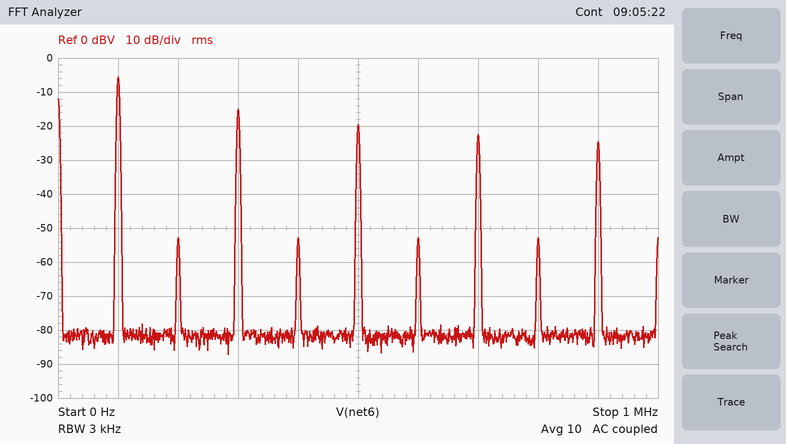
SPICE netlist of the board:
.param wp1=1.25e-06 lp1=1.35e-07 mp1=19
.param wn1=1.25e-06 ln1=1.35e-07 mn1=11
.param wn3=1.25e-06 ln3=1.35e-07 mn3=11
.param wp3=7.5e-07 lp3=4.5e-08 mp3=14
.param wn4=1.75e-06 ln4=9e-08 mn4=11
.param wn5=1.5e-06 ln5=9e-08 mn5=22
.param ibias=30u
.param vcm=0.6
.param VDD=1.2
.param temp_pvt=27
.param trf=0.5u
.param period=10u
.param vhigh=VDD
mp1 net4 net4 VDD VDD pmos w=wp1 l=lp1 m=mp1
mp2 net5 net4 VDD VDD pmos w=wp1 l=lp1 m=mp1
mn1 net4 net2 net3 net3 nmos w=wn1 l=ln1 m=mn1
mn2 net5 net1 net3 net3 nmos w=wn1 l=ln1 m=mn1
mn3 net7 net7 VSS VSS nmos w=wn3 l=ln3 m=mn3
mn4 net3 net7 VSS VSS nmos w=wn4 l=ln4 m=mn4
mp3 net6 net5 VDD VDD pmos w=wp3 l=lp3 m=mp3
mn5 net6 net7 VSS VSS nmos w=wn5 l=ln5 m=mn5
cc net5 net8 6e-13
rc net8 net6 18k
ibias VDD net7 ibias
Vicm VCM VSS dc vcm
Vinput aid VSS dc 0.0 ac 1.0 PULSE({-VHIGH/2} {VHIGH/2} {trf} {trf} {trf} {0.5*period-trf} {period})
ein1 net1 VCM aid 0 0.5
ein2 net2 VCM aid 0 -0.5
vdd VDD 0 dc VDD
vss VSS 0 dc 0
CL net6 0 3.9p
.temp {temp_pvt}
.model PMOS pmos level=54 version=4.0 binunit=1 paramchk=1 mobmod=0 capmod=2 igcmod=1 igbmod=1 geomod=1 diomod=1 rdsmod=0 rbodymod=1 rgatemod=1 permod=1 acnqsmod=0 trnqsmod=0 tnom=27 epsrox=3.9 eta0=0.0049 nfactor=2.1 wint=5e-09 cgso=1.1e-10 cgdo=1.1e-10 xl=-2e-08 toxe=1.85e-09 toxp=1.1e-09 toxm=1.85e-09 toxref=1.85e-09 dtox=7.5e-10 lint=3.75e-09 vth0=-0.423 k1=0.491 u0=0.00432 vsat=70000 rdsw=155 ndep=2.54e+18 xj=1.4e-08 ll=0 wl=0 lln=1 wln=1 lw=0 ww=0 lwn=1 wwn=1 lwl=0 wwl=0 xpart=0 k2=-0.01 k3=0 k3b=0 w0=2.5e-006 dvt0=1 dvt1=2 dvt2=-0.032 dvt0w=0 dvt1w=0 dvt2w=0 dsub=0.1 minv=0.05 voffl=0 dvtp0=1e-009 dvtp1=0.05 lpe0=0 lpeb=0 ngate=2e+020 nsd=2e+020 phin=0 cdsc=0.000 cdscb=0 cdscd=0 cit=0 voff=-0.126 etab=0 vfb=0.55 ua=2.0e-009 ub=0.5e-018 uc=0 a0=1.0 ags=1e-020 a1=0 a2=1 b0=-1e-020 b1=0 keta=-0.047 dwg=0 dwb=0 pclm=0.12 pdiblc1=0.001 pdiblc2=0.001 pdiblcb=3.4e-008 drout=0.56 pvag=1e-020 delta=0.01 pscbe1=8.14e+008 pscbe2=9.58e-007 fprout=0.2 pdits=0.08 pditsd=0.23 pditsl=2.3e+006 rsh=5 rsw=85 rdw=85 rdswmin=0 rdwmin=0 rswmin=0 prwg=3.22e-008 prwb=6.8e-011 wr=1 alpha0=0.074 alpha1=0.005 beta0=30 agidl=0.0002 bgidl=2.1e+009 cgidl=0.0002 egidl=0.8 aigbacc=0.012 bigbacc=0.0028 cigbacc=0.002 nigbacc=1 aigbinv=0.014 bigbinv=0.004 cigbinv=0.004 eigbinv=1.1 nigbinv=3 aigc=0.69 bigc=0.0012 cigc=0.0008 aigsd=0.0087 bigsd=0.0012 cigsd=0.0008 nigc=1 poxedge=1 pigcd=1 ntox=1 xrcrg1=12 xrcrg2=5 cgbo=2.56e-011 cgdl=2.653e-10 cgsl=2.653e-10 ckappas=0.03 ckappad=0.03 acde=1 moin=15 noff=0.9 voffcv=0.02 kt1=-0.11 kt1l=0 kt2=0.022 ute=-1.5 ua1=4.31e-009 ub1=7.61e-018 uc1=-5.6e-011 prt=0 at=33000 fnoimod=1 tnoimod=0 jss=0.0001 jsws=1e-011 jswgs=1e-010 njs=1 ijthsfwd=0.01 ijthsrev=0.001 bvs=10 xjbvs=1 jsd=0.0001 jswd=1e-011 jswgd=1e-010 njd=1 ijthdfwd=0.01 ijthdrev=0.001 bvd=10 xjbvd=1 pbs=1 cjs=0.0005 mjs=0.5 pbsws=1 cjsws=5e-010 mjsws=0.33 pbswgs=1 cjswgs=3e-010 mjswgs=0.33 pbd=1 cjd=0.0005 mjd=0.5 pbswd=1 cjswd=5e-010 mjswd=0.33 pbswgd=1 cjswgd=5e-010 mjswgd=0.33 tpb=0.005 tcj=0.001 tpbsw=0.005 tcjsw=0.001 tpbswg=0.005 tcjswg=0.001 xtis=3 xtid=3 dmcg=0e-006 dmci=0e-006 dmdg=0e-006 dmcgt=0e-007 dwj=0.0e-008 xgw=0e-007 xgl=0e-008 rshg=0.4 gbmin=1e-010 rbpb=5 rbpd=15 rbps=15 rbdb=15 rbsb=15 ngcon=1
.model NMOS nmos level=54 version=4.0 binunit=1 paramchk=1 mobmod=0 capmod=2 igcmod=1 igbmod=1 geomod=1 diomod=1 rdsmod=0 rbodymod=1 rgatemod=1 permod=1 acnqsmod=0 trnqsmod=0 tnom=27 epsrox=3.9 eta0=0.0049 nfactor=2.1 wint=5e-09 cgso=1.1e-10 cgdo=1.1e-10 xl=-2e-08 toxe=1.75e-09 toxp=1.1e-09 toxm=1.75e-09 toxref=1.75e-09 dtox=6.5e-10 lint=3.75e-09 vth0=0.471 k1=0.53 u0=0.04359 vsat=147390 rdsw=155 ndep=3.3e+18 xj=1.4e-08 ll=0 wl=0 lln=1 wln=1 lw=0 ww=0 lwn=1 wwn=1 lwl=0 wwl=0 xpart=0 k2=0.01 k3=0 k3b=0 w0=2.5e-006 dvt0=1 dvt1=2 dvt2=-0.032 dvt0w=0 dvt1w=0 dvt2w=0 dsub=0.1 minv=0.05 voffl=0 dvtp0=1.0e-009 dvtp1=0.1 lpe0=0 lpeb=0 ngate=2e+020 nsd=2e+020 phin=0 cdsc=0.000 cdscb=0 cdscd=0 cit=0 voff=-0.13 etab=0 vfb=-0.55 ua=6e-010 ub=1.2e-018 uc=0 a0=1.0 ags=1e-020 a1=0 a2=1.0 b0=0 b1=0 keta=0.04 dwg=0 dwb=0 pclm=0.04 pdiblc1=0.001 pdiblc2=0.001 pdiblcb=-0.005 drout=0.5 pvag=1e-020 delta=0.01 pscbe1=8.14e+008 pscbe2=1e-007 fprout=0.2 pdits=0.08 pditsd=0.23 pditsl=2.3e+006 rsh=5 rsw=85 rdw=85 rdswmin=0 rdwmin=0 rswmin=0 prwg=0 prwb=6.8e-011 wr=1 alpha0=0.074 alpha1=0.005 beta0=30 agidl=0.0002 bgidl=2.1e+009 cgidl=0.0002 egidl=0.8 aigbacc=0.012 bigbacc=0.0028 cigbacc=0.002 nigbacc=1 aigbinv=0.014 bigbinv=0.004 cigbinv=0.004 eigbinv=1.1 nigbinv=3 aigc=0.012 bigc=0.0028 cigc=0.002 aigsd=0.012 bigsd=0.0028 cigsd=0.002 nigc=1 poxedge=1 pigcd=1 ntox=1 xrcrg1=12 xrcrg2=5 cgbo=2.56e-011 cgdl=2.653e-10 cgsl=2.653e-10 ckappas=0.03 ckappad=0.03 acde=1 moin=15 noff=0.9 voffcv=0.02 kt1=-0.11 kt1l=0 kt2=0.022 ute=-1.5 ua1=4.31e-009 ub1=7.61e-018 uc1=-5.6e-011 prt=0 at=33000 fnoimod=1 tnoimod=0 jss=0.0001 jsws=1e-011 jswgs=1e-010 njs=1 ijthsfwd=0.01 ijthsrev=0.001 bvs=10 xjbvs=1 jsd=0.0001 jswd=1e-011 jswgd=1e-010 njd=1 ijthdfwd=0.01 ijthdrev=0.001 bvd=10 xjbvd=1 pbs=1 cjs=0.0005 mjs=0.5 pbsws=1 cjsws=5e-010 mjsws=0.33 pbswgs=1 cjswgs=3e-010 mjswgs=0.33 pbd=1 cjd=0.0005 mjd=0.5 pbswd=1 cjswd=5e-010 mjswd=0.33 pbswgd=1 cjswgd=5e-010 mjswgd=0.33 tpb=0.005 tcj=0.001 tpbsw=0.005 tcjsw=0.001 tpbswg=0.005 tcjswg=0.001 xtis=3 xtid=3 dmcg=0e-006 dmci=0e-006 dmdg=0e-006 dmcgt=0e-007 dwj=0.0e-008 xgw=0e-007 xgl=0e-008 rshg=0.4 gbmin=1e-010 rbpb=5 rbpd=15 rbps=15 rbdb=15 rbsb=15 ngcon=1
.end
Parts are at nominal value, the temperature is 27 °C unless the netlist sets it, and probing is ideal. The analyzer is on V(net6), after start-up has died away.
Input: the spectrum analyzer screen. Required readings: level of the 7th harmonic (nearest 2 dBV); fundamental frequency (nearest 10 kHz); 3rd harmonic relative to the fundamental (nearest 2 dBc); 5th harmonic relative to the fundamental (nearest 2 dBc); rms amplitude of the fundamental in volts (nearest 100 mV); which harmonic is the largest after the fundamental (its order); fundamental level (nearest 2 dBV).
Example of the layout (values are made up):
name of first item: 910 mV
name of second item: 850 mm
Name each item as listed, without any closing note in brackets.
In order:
level of the 7th harmonic: -22 dBV
fundamental frequency: 100 kHz
3rd harmonic relative to the fundamental: -10 dBc
5th harmonic relative to the fundamental: -14 dBc
rms amplitude of the fundamental in volts: 500 mV
which harmonic is the largest after the fundamental: 3
fundamental level: -6 dBV
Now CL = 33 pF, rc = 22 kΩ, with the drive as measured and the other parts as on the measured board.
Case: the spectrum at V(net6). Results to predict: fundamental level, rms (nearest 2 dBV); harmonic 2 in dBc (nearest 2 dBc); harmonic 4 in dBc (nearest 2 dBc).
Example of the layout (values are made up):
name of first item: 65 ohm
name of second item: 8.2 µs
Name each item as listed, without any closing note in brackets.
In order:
fundamental level, rms: -6 dBV
harmonic 2 in dBc: -28 dBc
harmonic 4 in dBc: -28 dBc
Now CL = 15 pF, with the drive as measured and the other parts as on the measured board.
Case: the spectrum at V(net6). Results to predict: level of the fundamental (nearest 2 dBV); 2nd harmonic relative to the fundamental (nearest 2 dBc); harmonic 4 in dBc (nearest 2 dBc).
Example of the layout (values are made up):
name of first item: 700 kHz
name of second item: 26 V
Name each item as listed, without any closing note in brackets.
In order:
level of the fundamental: -6 dBV
2nd harmonic relative to the fundamental: -36 dBc
harmonic 4 in dBc: -36 dBc
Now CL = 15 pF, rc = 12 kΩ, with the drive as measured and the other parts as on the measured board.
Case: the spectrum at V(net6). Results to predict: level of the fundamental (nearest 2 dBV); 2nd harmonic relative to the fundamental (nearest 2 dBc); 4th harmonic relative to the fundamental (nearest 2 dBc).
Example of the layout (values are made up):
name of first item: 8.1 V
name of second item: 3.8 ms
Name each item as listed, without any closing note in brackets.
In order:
level of the fundamental: -6 dBV
2nd harmonic relative to the fundamental: -36 dBc
4th harmonic relative to the fundamental: -36 dBc
